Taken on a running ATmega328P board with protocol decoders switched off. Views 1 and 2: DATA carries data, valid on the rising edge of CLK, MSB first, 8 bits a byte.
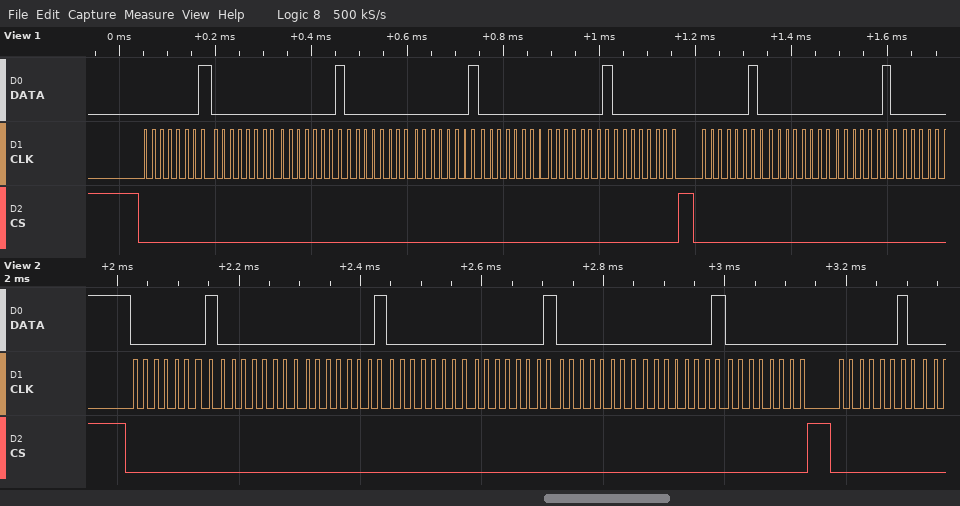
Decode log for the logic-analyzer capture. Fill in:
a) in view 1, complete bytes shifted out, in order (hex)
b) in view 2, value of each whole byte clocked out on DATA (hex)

01 00 01 00 01 00 01 00 02 00 02
0x01 0x00 0x01 0x00 0x01 0x00 0x01 0x00 0x02
